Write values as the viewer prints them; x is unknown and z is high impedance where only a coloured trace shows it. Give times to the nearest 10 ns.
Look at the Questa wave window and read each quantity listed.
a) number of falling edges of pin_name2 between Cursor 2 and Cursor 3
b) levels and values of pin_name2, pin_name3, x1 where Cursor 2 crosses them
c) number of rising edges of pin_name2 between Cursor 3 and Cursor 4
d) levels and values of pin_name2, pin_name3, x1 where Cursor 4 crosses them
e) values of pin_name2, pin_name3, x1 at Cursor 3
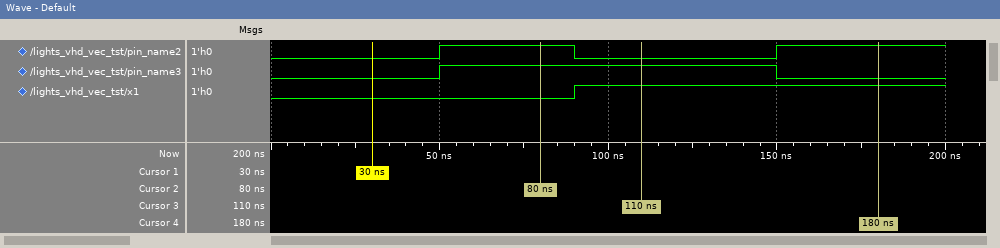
1
pin_name2=1, pin_name3=1, x1=0
1
pin_name2=1, pin_name3=0, x1=1
pin_name2=0, pin_name3=1, x1=1
